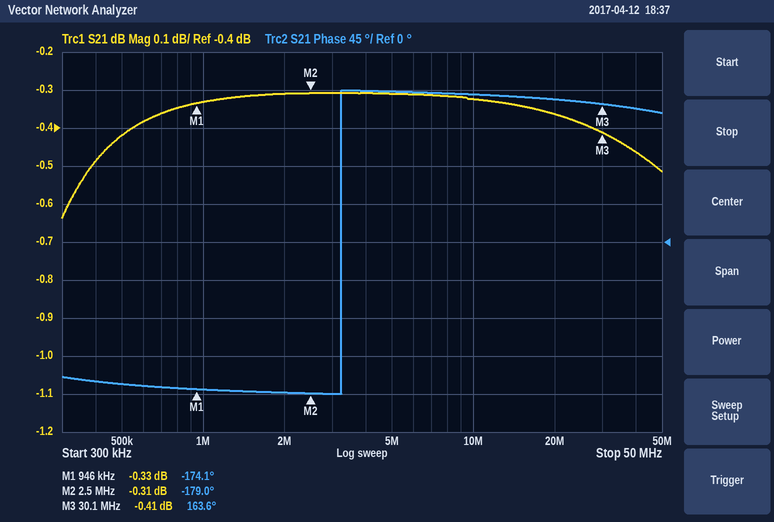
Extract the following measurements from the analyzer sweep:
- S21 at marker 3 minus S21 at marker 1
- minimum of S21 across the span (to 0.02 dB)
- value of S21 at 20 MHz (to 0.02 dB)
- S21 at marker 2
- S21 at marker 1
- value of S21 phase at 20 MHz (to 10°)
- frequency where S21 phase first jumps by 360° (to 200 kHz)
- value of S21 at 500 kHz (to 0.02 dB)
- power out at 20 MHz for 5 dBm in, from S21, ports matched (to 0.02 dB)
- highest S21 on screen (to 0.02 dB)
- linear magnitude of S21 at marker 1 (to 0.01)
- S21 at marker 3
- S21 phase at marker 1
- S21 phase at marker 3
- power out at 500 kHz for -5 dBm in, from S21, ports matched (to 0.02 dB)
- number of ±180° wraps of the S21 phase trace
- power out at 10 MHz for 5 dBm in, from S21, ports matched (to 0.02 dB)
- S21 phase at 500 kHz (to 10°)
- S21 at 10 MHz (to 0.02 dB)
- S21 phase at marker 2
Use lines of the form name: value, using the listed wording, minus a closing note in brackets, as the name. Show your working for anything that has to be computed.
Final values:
S21 at marker 3 minus S21 at marker 1: -0.41 − (-0.33) = -0.08 dB
minimum of S21 across the span: -0.64 dB
value of S21 at 20 MHz: -0.36 dB
S21 at marker 2: -0.31 dB
S21 at marker 1: -0.33 dB
value of S21 phase at 20 MHz: 170°
frequency where S21 phase first jumps by 360°: 3.2 MHz
value of S21 at 500 kHz: -0.42 dB
power out at 20 MHz for 5 dBm in, from S21, ports matched: 5 dBm + (-0.36 dB) = 4.64 dBm
highest S21 on screen: -0.30 dB
linear magnitude of S21 at marker 1: 10^(-0.33/20) ≈ 0.96
S21 at marker 3: -0.41 dB
S21 phase at marker 1: -174.1°
S21 phase at marker 3: 163.6°
power out at 500 kHz for -5 dBm in, from S21, ports matched: -5 dBm + (-0.42 dB) = -5.42 dBm
number of ±180° wraps of the S21 phase trace: 1
power out at 10 MHz for 5 dBm in, from S21, ports matched: 5 dBm + (-0.32 dB) = 4.68 dBm
S21 phase at 500 kHz: -170°
S21 at 10 MHz: -0.32 dB
S21 phase at marker 2: -179.0°
